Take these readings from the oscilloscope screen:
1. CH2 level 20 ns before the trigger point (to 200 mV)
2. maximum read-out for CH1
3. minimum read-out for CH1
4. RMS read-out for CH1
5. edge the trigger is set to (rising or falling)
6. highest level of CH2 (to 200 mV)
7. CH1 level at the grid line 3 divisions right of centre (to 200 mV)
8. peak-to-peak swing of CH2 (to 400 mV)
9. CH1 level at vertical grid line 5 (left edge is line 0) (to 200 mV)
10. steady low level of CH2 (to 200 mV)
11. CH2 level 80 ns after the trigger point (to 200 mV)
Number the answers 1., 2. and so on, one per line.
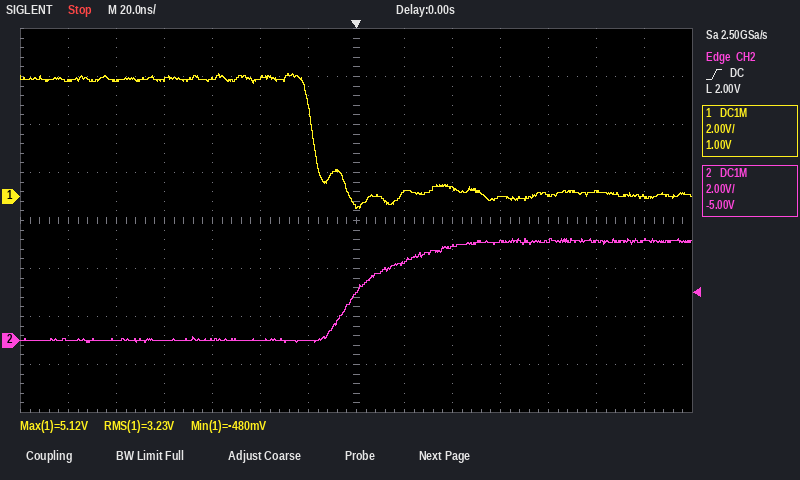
1. 0.0 V
2. 5.12 V
3. -480 mV
4. 3.23 V
5. rising
6. 4.2 V
7. 0.0 V
8. 4.4 V
9. 5.0 V
10. 0.0 V
11. 4.2 V
